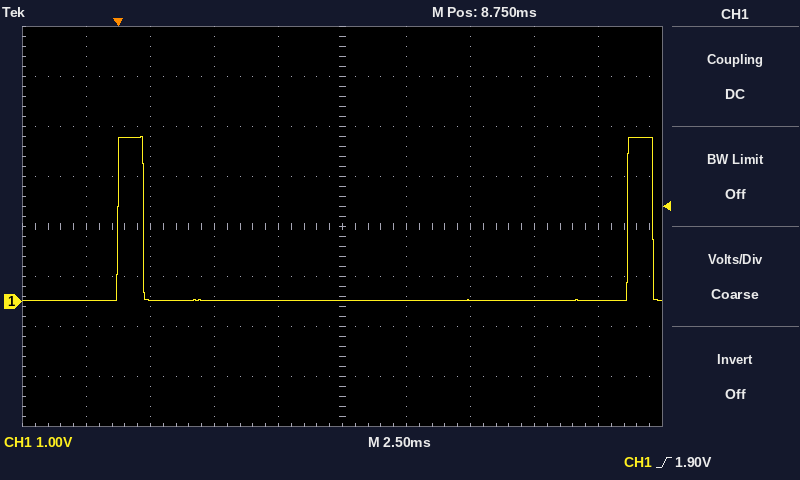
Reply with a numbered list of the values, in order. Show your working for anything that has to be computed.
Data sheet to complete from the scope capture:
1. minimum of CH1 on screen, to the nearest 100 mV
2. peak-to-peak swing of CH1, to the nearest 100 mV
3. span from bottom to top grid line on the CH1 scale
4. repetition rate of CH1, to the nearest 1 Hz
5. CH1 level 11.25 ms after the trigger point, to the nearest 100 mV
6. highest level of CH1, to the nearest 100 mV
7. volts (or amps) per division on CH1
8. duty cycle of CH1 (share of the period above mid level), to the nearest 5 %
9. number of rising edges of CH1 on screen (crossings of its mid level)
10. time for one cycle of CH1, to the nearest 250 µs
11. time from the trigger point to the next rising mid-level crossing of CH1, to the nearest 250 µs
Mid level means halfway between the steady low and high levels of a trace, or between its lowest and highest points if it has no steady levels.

1. 0.0 V
2. 3.3 V − (0.0 V) = 3.3 V
3. 8 V
4. 1 / 20.00 ms ≈ 50 Hz
5. 0.0 V
6. 3.3 V
7. 1 V
8. 5 %
9. 2
10. 20.00 ms
11. 20.00 ms
